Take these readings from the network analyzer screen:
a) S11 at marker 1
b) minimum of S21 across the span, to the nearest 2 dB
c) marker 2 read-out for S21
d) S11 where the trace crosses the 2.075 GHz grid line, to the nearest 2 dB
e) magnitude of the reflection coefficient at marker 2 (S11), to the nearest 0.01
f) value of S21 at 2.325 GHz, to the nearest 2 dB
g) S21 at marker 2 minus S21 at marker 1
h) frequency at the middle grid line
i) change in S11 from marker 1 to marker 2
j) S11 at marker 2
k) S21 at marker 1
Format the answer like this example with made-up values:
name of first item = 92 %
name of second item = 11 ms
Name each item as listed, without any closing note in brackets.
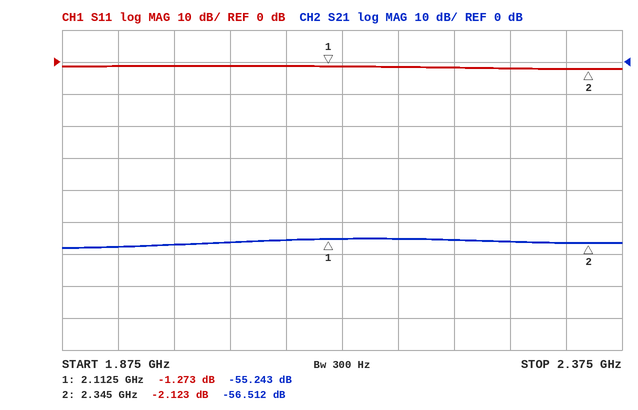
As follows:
S11 at marker 1 = -1.273 dB
minimum of S21 across the span, to the nearest 2 dB = -58 dB
marker 2 read-out for S21 = -56.512 dB
S11 where the trace crosses the 2.075 GHz grid line, to the nearest 2 dB = -2 dB
magnitude of the reflection coefficient at marker 2 (S11), to the nearest 0.01 = 0.78
value of S21 at 2.325 GHz, to the nearest 2 dB = -56 dB
S21 at marker 2 minus S21 at marker 1 = -1.269 dB
frequency at the middle grid line = 2.125 GHz
change in S11 from marker 1 to marker 2 = -0.850 dB
S11 at marker 2 = -2.123 dB
S21 at marker 1 = -55.243 dB
